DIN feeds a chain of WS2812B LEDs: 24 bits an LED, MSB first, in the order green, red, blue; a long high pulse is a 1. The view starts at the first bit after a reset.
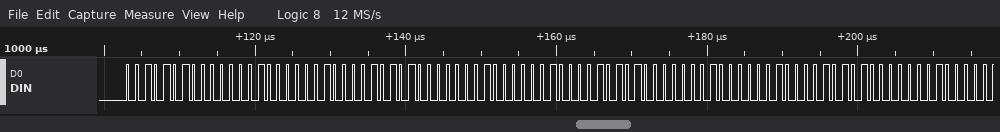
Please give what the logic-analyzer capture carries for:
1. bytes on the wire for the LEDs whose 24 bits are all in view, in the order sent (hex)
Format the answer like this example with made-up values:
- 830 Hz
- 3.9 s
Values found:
- 2A 02 04 2A 02 04 2A 02 04
